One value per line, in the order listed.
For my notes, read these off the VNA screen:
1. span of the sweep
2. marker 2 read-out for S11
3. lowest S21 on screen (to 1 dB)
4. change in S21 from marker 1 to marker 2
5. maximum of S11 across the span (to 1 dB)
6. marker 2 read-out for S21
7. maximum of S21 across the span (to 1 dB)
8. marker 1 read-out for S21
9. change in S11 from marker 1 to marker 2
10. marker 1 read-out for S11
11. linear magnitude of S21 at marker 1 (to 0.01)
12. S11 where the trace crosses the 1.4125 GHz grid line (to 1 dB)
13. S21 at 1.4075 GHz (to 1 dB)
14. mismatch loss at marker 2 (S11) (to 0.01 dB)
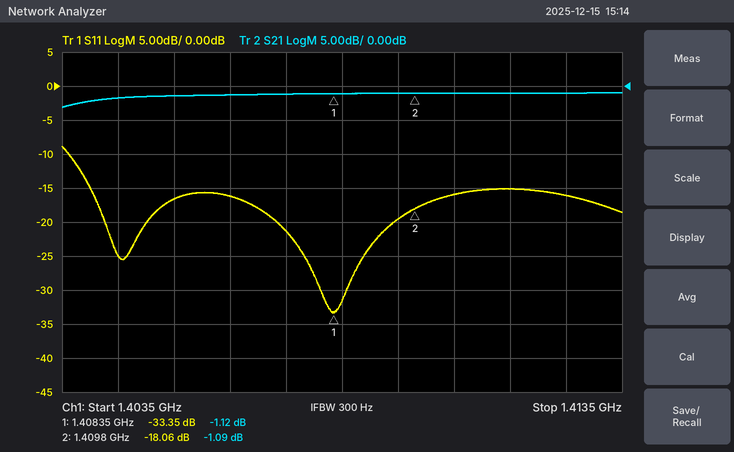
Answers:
10 MHz
-18.06 dB
-3 dB
0.03 dB
-9 dB
-1.09 dB
-1 dB
-1.12 dB
15.29 dB
-33.35 dB
0.88
-16 dB
-1 dB
0.07 dB
